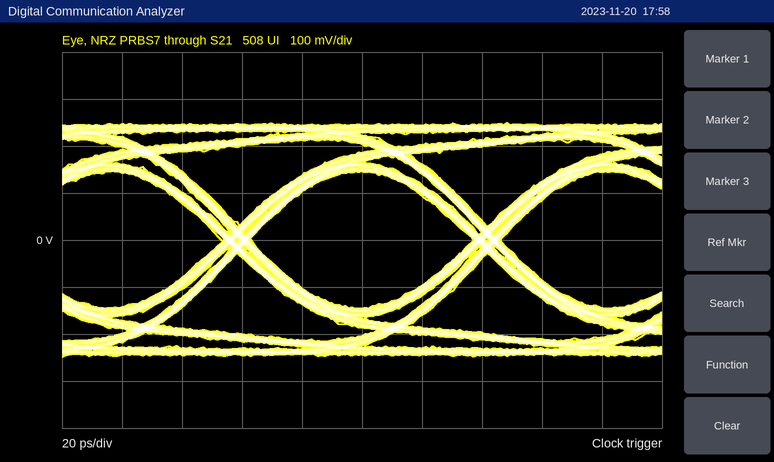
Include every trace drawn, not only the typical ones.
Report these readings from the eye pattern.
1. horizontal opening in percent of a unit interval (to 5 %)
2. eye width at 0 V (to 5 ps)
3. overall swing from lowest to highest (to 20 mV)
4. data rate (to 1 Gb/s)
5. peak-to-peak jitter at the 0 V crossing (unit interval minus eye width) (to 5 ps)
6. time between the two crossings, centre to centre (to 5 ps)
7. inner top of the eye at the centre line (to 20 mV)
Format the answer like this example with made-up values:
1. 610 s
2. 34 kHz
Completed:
1. 90 %
2. 75 ps
3. 500 mV
4. 12 Gb/s
5. 10 ps
6. 85 ps
7. 140 mV
